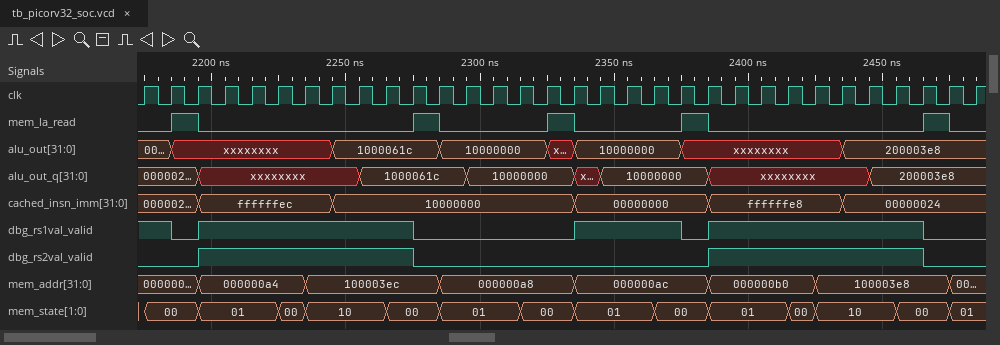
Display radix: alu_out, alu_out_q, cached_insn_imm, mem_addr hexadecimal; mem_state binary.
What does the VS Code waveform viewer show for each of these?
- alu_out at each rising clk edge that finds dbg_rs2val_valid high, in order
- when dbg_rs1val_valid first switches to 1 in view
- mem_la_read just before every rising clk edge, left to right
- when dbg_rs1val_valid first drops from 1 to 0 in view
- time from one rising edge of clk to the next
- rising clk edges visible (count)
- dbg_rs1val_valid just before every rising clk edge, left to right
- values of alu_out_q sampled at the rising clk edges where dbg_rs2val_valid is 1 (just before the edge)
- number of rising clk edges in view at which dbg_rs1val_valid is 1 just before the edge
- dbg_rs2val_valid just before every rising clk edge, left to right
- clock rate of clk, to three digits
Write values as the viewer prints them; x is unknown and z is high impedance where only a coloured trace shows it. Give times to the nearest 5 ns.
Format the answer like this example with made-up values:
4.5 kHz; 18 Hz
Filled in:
xxxxxxxx, xxxxxxxx, xxxxxxxx, xxxxxxxx, xxxxxxxx, 1000061c, 1000061c, 1000061c, xxxxxxxx, xxxxxxxx, xxxxxxxx, xxxxxxxx, xxxxxxxx, 200003e8, 200003e8, 200003e8; 2195 ns; 0 0 1 0 0 0 0 0 0 0 0 1 0 0 0 0 1 0 0 0 0 1 0 0 0 0 0 0 0 0 1 0; 2185 ns; 10 ns; 32; 1 1 0 1 1 1 1 1 1 1 1 0 0 0 0 0 0 1 1 1 1 0 1 1 1 1 1 1 1 1 0 0; xxxxxxxx, xxxxxxxx, xxxxxxxx, xxxxxxxx, xxxxxxxx, xxxxxxxx, 1000061c, 1000061c, xxxxxxxx, xxxxxxxx, xxxxxxxx, xxxxxxxx, xxxxxxxx, xxxxxxxx, 200003e8, 200003e8; 22; 0 0 0 1 1 1 1 1 1 1 1 0 0 0 0 0 0 0 0 0 0 0 1 1 1 1 1 1 1 1 0 0; 100 MHz
